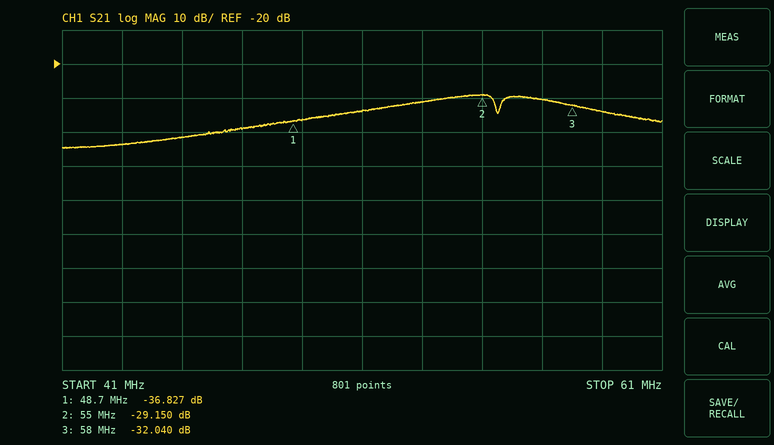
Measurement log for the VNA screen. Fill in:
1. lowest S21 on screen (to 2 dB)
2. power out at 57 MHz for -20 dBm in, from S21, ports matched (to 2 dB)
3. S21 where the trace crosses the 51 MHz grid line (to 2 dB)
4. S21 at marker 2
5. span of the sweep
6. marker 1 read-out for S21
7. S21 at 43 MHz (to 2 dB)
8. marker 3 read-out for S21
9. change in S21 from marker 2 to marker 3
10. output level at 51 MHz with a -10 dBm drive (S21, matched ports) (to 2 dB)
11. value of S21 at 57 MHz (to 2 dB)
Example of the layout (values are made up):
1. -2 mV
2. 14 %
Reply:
1. -44 dB
2. -50 dBm
3. -34 dB
4. -29.150 dB
5. 20 MHz
6. -36.827 dB
7. -44 dB
8. -32.040 dB
9. -2.890 dB
10. -44 dBm
11. -30 dB
